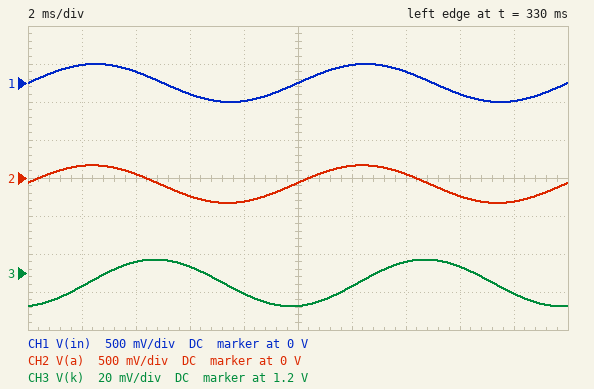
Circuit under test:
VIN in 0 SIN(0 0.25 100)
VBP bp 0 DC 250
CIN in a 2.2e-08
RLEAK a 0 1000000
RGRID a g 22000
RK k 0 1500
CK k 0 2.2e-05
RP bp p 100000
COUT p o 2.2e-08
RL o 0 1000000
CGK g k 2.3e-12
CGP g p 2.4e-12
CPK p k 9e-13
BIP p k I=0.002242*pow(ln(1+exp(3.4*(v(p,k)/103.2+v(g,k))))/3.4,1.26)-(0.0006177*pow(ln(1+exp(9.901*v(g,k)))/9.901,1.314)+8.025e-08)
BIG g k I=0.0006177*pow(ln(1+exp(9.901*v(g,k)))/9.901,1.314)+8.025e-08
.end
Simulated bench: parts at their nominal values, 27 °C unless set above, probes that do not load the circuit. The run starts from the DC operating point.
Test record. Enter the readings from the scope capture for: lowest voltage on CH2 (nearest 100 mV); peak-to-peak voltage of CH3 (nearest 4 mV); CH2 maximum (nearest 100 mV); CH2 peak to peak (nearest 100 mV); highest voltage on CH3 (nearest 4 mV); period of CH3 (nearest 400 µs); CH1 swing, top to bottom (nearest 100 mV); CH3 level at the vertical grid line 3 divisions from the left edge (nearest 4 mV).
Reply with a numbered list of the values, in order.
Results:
1. -300 mV
2. 24 mV
3. 200 mV
4. 500 mV
5. 1.208 V
6. 10.0 ms
7. 500 mV
8. 1.204 V
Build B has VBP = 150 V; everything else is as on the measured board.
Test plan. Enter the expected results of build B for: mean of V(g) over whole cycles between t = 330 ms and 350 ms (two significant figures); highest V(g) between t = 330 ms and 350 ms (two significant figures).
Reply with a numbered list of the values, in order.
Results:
1. -86 mV
2. 160 mV
